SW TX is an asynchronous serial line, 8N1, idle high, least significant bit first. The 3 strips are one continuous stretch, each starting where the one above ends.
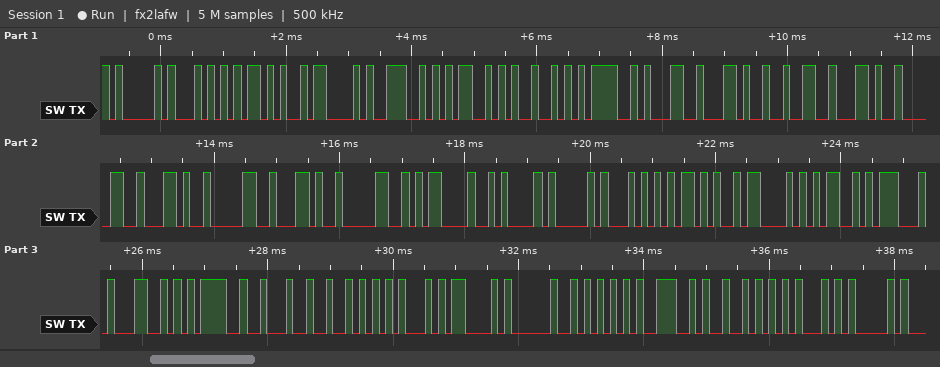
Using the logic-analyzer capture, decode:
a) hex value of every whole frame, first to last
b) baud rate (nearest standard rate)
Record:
41 54 2B 43 4E 4D 49 3D 31 2C 32 2C 30 2C 30 2C 30 0D 0A 41 54 2B 43 4D 47 4C 3D 22 52 45 43 20 55 4E 52 45 41
9600 baud
